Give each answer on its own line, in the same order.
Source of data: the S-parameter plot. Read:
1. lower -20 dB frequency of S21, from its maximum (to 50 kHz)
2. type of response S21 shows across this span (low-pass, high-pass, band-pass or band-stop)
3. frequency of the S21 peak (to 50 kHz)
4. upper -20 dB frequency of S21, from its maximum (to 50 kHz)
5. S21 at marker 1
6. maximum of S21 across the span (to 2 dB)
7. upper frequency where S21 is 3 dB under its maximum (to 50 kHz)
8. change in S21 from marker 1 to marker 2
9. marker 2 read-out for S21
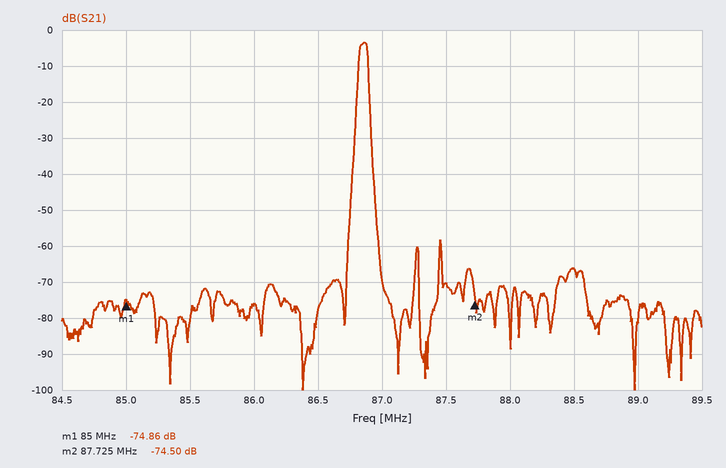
86.80 MHz
band-pass
86.85 MHz
86.90 MHz
-74.86 dB
-4 dB
86.90 MHz
0.36 dB
-74.50 dB
